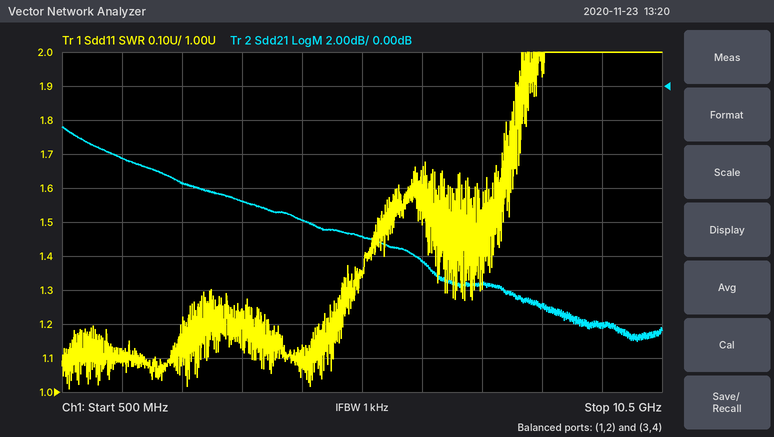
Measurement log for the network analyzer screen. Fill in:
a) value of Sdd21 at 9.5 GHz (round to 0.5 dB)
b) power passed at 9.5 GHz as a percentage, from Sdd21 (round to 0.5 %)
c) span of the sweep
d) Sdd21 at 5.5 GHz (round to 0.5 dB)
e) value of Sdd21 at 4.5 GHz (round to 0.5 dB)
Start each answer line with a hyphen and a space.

- -14.0 dB
- 4.0 %
- 10 GHz
- -9.0 dB
- -8.0 dB
